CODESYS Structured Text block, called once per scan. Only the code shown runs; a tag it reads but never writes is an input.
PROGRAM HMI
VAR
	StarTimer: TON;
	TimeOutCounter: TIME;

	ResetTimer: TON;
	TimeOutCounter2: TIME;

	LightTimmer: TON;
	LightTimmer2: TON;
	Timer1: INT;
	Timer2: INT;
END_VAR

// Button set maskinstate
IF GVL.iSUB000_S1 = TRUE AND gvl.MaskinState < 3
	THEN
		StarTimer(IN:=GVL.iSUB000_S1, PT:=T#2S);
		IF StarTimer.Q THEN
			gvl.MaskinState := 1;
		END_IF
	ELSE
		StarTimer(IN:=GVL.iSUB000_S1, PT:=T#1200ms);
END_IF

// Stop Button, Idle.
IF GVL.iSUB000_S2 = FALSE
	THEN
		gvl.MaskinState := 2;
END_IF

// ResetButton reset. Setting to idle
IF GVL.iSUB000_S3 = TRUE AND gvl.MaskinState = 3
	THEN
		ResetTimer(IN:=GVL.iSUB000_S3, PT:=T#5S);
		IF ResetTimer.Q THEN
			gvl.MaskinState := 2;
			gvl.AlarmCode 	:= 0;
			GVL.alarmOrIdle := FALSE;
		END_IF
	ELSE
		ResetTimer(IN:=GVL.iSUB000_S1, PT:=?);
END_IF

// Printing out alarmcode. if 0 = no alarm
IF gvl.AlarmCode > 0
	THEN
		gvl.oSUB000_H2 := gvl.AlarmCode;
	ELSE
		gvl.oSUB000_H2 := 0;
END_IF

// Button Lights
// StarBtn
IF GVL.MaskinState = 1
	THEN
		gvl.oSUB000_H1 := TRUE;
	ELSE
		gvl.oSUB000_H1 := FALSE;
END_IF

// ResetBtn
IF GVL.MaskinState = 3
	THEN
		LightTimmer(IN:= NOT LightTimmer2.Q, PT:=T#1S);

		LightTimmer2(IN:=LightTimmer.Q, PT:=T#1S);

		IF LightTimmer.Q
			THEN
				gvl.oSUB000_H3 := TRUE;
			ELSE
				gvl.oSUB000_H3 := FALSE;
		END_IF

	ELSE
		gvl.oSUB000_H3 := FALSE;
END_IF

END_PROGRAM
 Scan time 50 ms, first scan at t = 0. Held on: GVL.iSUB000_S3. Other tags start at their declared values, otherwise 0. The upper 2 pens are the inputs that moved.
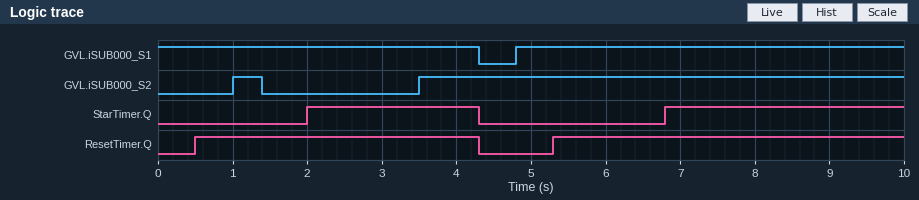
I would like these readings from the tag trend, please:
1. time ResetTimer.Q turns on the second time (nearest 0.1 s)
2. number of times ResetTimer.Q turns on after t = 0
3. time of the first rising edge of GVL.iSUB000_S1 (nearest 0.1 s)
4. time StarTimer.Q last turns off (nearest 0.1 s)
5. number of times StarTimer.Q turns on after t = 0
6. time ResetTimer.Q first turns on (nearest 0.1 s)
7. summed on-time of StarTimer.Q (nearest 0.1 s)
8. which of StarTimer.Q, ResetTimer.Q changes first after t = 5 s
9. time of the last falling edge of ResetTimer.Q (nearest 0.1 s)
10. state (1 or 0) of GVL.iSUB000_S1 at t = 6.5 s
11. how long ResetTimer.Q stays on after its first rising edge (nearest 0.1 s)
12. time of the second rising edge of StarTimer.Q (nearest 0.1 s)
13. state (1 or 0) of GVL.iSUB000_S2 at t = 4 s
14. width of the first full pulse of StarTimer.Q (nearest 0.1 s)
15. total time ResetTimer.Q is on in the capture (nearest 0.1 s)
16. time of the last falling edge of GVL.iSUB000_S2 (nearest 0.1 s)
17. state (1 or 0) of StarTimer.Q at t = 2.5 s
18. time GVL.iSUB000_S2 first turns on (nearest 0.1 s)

5.3 s
2
4.8 s
4.3 s
2
0.5 s
5.5 s
ResetTimer.Q
4.3 s
1
3.8 s
6.8 s
1
2.3 s
8.5 s
1.4 s
1
1.0 s
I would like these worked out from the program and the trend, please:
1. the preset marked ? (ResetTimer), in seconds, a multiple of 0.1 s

0.5 s
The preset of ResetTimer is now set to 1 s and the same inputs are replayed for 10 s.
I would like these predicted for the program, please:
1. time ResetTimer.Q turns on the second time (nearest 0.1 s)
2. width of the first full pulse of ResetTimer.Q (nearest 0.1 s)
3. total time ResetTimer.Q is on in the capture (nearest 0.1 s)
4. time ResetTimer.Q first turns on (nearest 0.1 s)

5.8 s
3.3 s
7.5 s
1.0 s
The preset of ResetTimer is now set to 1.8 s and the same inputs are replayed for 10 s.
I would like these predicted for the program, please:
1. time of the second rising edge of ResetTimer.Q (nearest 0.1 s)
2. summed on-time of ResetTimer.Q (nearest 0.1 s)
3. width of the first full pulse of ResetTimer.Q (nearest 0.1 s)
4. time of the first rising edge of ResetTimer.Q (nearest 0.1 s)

6.6 s
5.9 s
2.5 s
1.8 s
